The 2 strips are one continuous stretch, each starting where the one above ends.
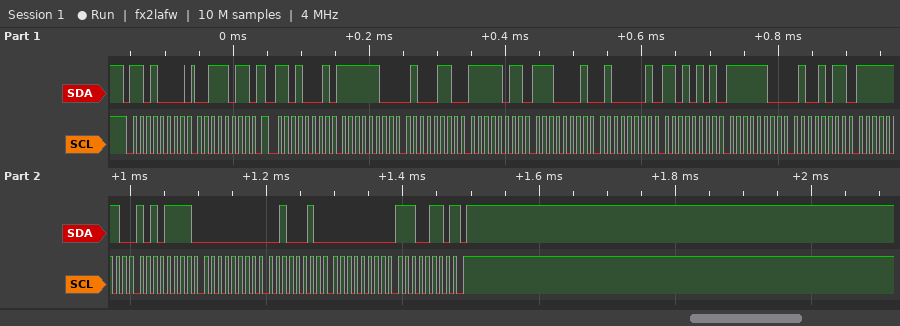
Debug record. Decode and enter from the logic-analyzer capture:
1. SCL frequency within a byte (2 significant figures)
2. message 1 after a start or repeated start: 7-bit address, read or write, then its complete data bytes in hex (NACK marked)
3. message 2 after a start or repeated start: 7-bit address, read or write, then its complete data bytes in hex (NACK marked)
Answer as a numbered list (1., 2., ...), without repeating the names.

1. 100 kHz
2. 0x68 write: 3B
3. 0x68 read: FC 46 FB E1 41 D5 FC 4B FE AF 00 22 00 E6 NACK
